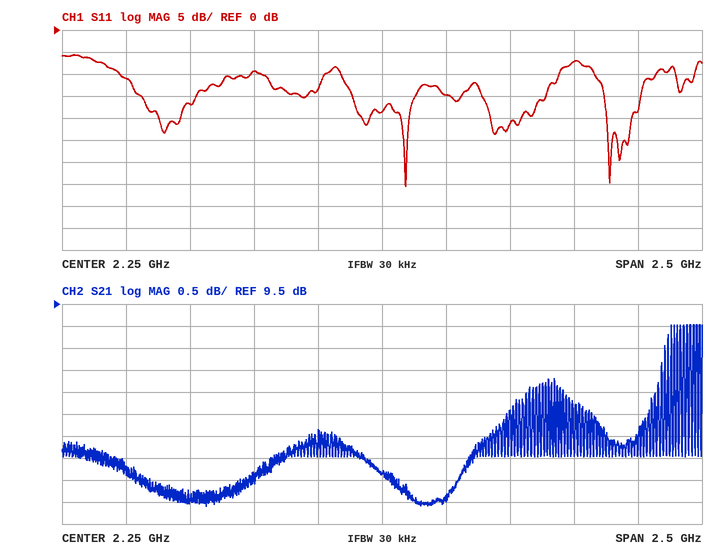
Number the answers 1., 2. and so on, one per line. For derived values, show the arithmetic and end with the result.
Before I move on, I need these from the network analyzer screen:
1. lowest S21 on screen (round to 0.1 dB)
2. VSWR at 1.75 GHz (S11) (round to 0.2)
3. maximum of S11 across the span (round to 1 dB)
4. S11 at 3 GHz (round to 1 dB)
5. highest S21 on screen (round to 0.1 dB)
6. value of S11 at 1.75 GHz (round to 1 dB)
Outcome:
1. 4.9 dB
2. |Γ| = 10^(-9/20) = 0.3548; VSWR = (1 + 0.3548)/(1 − 0.3548) ≈ 2.10, so 2.0 to the nearest 0.2
3. -6 dB
4. -7 dB
5. 9.0 dB
6. -9 dB
